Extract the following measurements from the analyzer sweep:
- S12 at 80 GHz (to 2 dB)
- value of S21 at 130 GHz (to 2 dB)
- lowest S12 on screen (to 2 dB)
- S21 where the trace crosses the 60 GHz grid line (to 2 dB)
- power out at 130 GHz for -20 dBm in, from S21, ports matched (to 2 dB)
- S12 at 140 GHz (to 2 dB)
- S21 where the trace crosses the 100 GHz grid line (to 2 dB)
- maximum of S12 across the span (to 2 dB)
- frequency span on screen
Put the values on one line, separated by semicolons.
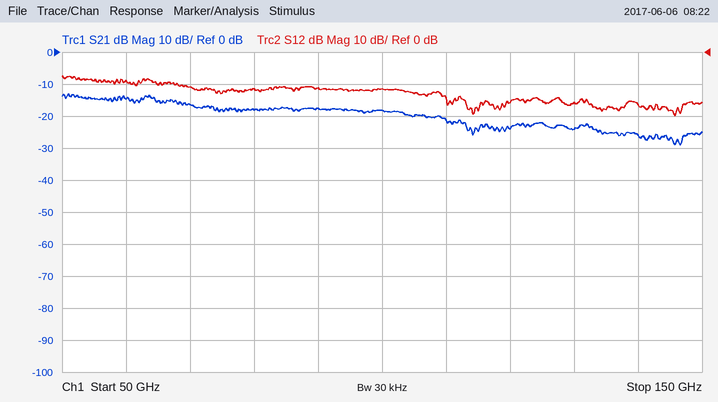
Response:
-12 dB; -24 dB; -20 dB; -14 dB; -44 dBm; -16 dB; -18 dB; -8 dB; 100 GHz
